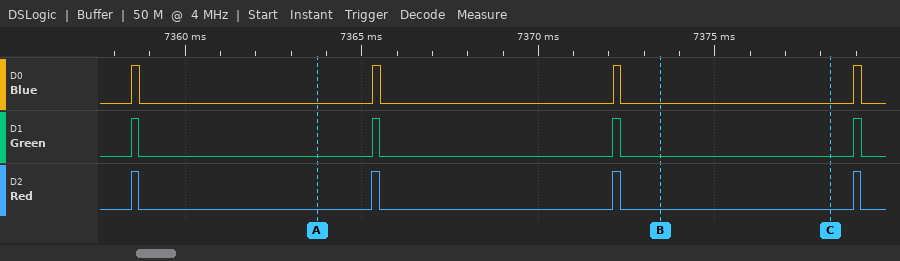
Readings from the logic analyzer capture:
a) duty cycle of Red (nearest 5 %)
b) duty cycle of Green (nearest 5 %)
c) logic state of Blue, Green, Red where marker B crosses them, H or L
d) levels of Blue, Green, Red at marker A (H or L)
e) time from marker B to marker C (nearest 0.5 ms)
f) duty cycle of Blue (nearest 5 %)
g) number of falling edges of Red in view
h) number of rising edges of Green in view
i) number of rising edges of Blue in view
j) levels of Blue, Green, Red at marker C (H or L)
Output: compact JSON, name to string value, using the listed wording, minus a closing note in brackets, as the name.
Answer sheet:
{"duty cycle of Red": "5 %", "duty cycle of Green": "5 %", "logic state of Blue, Green, Red where marker B crosses them, H or L": "Blue=L, Green=L, Red=L", "levels of Blue, Green, Red at marker A": "Blue=L, Green=L, Red=L", "time from marker B to marker C": "5 ms", "duty cycle of Blue": "5 %", "number of falling edges of Red in view": "4", "number of rising edges of Green in view": "4", "number of rising edges of Blue in view": "4", "levels of Blue, Green, Red at marker C": "Blue=L, Green=L, Red=L"}
